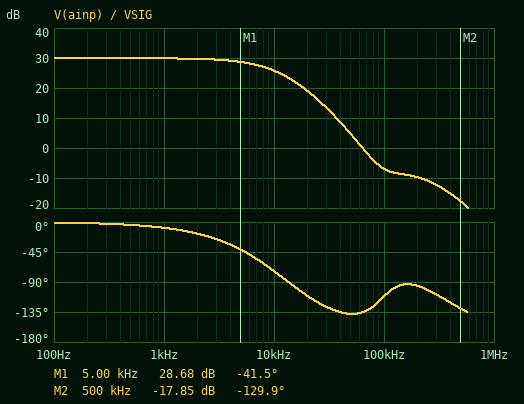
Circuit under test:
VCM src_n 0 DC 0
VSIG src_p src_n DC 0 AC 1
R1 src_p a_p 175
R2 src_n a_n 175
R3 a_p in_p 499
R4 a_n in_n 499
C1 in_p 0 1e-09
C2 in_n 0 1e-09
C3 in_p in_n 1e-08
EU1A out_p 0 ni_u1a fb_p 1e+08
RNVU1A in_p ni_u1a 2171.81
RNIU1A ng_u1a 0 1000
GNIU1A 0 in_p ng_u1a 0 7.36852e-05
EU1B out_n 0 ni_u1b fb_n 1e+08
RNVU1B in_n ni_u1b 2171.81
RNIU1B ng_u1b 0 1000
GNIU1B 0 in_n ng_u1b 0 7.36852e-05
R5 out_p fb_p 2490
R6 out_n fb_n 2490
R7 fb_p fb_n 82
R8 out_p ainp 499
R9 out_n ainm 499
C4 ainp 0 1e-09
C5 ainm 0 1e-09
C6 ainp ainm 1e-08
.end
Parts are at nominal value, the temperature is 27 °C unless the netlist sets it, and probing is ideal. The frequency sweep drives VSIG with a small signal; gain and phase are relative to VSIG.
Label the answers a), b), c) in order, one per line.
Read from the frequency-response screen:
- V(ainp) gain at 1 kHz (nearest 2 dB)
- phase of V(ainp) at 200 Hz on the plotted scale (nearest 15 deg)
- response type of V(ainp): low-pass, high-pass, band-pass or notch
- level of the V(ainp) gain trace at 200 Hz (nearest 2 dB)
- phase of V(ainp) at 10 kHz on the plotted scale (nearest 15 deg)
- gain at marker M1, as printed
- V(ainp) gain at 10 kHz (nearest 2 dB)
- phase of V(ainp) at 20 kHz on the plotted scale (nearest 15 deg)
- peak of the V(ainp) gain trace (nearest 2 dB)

a) 30 dB
b) 0 deg
c) low-pass
d) 30 dB
e) -75 deg
f) 28.68 dB
g) 26 dB
h) -105 deg
i) 30 dB
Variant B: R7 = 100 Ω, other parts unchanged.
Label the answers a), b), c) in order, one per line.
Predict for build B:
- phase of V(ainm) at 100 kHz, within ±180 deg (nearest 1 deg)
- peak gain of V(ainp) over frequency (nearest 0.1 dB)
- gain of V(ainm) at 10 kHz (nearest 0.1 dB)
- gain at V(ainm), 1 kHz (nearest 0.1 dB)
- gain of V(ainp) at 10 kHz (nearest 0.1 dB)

a) -13 deg
b) 28.3 dB
c) 23.9 dB
d) 27.9 dB
e) 24.1 dB
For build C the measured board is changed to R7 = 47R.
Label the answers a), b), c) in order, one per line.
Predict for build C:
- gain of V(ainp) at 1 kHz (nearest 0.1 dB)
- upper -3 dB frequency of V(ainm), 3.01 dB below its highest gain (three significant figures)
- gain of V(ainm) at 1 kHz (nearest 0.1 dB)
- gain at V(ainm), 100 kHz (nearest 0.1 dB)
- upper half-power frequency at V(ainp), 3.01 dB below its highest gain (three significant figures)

a) 34.6 dB
b) 8.32 kHz
c) 34.4 dB
d) 1.6 dB
e) 8.24 kHz
